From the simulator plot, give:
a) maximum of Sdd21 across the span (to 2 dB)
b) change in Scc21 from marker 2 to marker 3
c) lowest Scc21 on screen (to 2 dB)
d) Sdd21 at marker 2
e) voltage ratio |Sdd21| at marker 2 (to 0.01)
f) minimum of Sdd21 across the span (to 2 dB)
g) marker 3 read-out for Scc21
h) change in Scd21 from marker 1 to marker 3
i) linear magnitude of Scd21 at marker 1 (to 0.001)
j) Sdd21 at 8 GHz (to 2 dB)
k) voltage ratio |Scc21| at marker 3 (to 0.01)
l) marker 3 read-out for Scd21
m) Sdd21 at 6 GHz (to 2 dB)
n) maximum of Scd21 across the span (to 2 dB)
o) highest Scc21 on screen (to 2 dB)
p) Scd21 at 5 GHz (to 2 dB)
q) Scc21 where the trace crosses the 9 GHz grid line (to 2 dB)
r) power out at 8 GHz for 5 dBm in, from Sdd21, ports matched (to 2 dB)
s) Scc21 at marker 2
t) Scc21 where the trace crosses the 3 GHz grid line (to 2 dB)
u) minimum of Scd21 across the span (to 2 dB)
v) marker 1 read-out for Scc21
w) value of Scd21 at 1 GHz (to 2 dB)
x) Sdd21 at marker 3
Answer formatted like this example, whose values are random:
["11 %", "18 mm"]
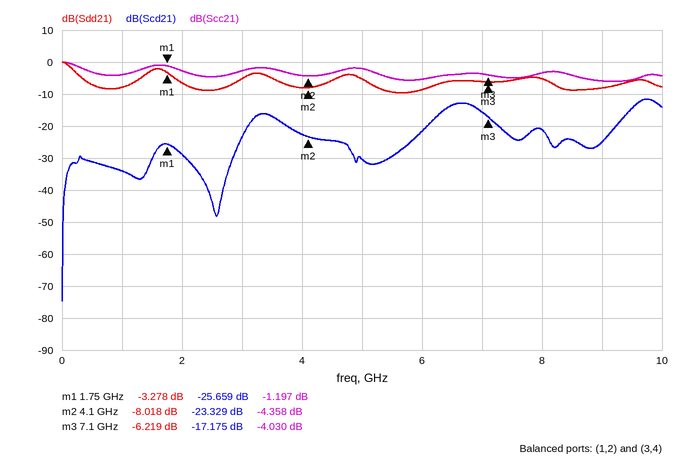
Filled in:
["0 dB", "0.328 dB", "-6 dB", "-8.018 dB", "0.40", "-10 dB", "-4.030 dB", "8.484 dB", "0.052", "-6 dB", "0.63", "-17.175 dB", "-8 dB", "-12 dB", "0 dB", "-30 dB", "-6 dB", "0 dBm", "-4.358 dB", "-2 dB", "-74 dB", "-1.197 dB", "-34 dB", "-6.219 dB"]
